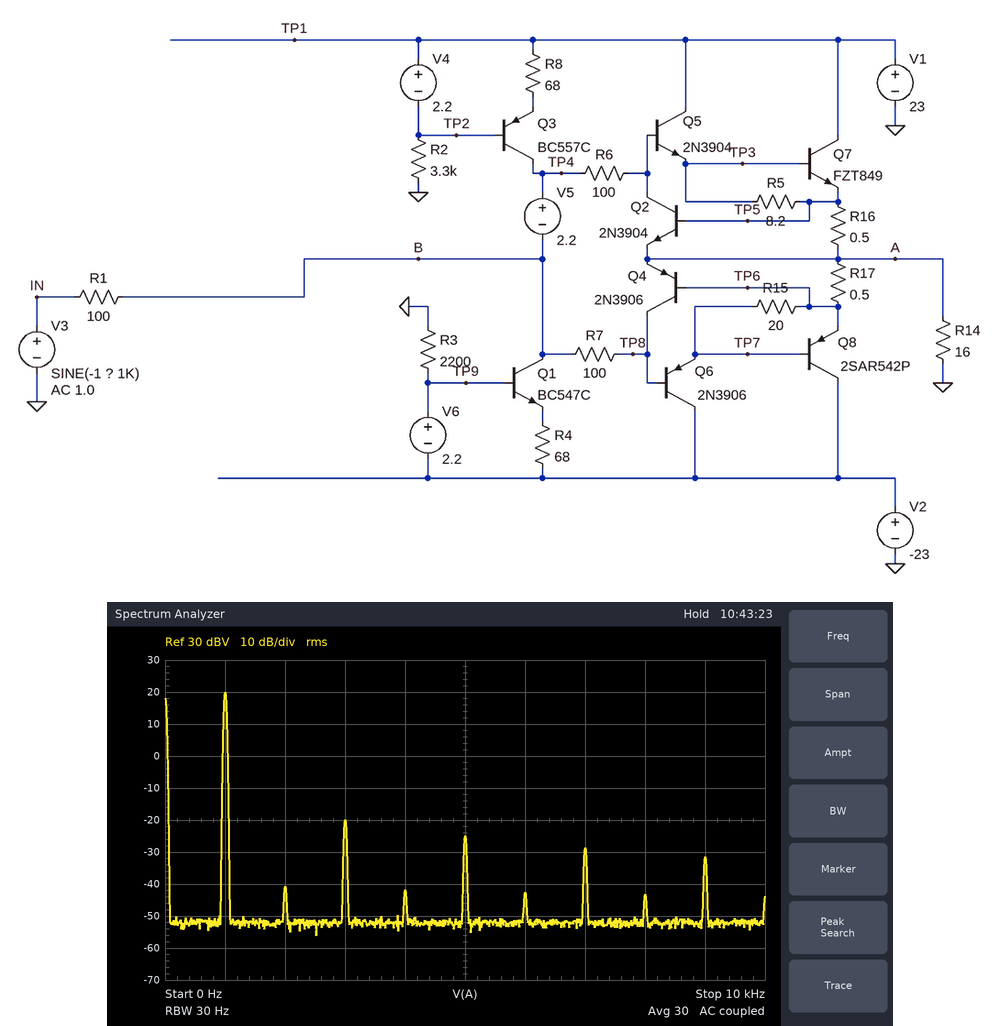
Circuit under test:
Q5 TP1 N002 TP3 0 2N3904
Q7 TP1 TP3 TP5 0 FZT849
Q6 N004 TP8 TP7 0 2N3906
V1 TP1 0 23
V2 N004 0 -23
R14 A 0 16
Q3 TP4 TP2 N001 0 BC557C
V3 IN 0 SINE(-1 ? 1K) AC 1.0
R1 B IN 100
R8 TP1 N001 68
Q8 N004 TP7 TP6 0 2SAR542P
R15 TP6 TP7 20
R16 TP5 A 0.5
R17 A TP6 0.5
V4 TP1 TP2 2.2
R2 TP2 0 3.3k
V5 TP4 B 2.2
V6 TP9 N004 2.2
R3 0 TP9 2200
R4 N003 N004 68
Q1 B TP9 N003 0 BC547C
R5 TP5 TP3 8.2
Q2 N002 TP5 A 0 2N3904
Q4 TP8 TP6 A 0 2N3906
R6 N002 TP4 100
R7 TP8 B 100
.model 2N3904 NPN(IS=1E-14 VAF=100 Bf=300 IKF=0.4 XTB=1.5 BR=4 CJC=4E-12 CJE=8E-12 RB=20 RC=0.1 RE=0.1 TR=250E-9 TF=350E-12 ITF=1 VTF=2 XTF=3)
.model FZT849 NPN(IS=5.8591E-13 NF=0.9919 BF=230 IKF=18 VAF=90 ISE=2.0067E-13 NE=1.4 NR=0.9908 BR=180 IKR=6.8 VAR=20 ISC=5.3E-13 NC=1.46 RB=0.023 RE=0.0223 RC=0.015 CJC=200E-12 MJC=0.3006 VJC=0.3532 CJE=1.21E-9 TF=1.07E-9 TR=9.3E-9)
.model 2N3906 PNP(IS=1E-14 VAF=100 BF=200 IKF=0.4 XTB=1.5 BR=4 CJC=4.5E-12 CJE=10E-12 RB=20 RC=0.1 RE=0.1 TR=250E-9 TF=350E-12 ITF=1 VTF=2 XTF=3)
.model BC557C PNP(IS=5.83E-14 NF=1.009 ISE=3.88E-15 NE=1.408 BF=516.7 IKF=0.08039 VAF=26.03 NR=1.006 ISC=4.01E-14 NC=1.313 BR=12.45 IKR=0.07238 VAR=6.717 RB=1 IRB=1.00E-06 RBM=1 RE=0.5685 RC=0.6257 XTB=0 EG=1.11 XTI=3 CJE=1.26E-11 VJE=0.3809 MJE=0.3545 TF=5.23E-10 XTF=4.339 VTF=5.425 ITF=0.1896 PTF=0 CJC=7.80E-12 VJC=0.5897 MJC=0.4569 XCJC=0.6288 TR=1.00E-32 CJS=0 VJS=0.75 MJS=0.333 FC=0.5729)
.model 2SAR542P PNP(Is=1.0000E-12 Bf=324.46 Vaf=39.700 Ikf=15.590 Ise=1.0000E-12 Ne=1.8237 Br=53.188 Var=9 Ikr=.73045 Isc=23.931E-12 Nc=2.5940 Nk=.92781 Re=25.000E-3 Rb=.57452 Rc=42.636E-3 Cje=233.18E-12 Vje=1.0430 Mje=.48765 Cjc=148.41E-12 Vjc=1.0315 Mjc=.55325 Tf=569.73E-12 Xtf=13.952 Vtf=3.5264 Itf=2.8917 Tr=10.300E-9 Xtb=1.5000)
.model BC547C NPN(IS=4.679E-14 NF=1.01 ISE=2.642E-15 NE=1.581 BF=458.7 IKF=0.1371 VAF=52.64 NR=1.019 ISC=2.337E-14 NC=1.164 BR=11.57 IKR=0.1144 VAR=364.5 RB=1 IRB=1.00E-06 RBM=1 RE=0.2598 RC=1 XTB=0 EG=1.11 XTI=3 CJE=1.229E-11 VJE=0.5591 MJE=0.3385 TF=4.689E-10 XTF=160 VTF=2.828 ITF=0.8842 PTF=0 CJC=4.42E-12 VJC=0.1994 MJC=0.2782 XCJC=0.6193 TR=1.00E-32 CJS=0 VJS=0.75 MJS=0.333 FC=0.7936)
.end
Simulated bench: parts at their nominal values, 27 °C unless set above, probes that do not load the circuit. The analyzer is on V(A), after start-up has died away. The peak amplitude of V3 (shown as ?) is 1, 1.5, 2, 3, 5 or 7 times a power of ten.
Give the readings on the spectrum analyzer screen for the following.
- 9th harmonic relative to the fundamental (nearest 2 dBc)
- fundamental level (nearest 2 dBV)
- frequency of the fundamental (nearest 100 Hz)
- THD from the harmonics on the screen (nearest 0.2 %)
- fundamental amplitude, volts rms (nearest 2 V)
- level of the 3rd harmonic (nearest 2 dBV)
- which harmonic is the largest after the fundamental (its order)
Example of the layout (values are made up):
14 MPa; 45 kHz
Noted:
-52 dBc; 20 dBV; 1.0 kHz; 1.2 %; 10 V; -20 dBV; 3
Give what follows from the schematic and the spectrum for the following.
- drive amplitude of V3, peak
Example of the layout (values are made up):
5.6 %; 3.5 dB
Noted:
15 V
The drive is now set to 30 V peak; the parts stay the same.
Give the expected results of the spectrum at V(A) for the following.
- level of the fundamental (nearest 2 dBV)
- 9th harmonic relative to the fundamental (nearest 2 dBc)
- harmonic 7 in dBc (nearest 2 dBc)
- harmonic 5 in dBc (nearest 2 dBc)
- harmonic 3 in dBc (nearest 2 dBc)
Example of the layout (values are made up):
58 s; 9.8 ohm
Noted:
24 dBV; -50 dBc; -32 dBc; -32 dBc; -18 dBc
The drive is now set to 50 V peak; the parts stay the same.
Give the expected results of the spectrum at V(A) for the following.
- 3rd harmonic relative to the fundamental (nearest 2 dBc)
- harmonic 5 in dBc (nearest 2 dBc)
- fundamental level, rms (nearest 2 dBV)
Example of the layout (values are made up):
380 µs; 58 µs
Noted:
-12 dBc; -22 dBc; 24 dBV
